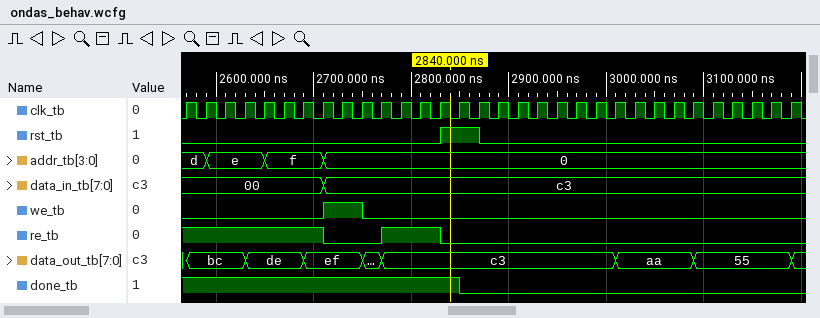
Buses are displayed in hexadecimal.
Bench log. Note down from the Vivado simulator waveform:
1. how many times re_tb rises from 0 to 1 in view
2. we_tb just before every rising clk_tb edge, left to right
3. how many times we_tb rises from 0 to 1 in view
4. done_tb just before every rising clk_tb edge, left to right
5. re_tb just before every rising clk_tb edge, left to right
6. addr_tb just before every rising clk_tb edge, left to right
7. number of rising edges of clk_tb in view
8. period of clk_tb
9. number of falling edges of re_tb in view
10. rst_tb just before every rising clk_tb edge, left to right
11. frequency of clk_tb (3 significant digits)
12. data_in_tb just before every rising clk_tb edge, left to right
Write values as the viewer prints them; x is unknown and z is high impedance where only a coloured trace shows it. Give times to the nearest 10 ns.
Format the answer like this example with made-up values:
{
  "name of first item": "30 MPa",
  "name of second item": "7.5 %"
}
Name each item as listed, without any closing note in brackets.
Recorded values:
{
  "how many times re_tb rises from 0 to 1 in view": "1",
  "we_tb just before every rising clk_tb edge, left to right": "0 0 0 0 0 0 0 0 1 1 0 0 0 0 0 0 0 0 0 0 0 0 0 0 0 0 0 0 0 0 0 0",
  "how many times we_tb rises from 0 to 1 in view": "1",
  "done_tb just before every rising clk_tb edge, left to right": "1 1 1 1 1 1 1 1 1 1 1 1 1 1 1 0 0 0 0 0 0 0 0 0 0 0 0 0 0 0 0 0",
  "re_tb just before every rising clk_tb edge, left to right": "1 1 1 1 1 1 1 1 0 0 0 1 1 1 0 0 0 0 0 0 0 0 0 0 0 0 0 0 0 0 0 0",
  "addr_tb just before every rising clk_tb edge, left to right": "d, d, e, e, e, f, f, f, 0, 0, 0, 0, 0, 0, 0, 0, 0, 0, 0, 0, 0, 0, 0, 0, 0, 0, 0, 0, 0, 0, 0, 0",
  "number of rising edges of clk_tb in view": "32",
  "period of clk_tb": "20 ns",
  "number of falling edges of re_tb in view": "2",
  "rst_tb just before every rising clk_tb edge, left to right": "0 0 0 0 0 0 0 0 0 0 0 0 0 0 1 1 0 0 0 0 0 0 0 0 0 0 0 0 0 0 0 0",
  "frequency of clk_tb": "50.0 MHz",
  "data_in_tb just before every rising clk_tb edge, left to right": "00, 00, 00, 00, 00, 00, 00, 00, c3, c3, c3, c3, c3, c3, c3, c3, c3, c3, c3, c3, c3, c3, c3, c3, c3, c3, c3, c3, c3, c3, c3, c3"
}
